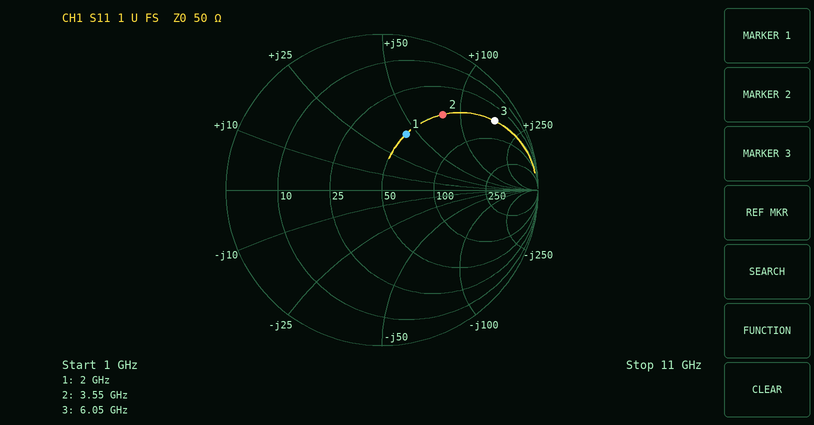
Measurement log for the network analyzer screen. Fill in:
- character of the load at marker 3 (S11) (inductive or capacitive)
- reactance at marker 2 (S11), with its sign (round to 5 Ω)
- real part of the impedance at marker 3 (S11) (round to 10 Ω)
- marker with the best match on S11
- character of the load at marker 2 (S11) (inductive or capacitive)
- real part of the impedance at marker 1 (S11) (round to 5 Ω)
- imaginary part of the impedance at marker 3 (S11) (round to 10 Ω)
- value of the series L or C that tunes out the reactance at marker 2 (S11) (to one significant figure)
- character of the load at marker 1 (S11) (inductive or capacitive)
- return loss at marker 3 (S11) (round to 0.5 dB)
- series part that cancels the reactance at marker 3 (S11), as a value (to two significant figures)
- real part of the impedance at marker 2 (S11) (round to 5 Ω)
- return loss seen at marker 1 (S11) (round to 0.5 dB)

inductive
+80 Ω
50 Ω
marker 1
inductive
50 Ω
+160 Ω
600 fF
inductive
1.5 dB
160 fF
50 Ω
8.0 dB
